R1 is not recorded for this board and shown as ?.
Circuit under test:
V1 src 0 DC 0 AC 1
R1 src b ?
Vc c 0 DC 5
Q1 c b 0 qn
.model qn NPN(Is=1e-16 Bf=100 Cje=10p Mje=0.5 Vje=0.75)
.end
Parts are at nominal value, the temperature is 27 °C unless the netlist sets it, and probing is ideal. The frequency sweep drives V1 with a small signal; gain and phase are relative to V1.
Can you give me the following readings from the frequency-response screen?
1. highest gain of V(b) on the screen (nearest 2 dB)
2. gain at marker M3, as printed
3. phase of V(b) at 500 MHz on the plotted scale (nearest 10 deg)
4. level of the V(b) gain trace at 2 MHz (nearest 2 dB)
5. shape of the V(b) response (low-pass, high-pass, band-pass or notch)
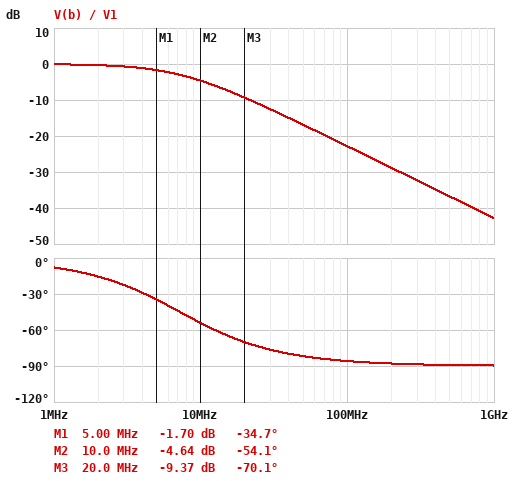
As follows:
0 dB
-9.37 dB
-90 deg
0 dB
low-pass
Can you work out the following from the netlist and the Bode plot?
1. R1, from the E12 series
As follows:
2.2 kΩ
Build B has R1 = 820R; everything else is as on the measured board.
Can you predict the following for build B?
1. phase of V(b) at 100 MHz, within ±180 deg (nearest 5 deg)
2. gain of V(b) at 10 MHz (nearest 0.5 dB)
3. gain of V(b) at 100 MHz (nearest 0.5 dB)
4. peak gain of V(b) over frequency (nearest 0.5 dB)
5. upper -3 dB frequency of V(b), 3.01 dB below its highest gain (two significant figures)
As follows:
-80 deg
-1.0 dB
-14.5 dB
0 dB
19 MHz
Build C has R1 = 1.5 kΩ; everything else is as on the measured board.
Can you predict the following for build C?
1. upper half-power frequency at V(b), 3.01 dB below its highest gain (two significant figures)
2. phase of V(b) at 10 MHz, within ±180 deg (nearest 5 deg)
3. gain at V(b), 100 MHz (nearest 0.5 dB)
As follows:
11 MHz
-45 deg
-19.5 dB
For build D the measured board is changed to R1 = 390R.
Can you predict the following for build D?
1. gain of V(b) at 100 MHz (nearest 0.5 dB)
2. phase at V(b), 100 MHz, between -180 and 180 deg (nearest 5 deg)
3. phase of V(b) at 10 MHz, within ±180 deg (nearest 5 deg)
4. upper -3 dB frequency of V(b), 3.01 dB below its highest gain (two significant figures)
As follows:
-8.5 dB
-70 deg
-15 deg
41 MHz
